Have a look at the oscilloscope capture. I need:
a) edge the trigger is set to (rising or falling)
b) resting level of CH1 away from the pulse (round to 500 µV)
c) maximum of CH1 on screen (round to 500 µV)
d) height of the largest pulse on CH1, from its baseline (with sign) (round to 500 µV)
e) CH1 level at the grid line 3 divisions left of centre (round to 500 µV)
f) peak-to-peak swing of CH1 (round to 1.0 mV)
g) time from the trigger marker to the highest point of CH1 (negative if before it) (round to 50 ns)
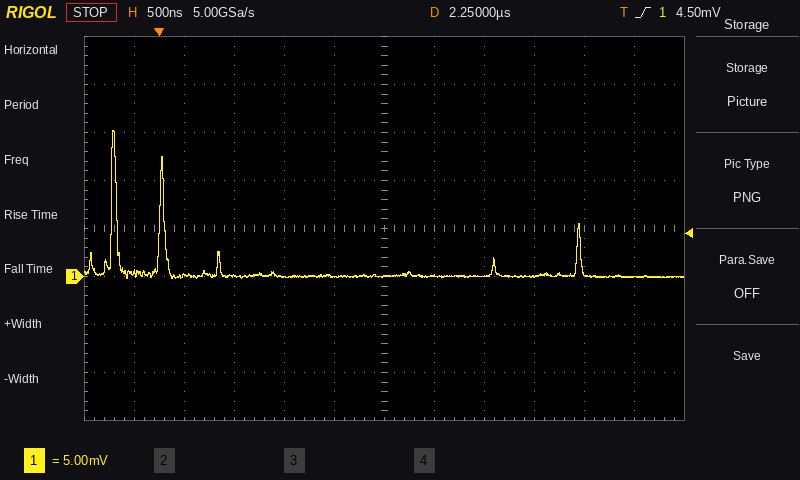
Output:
rising
0.0 mV
15.0 mV
+15.0 mV
0.0 mV
15.0 mV
-450 ns
